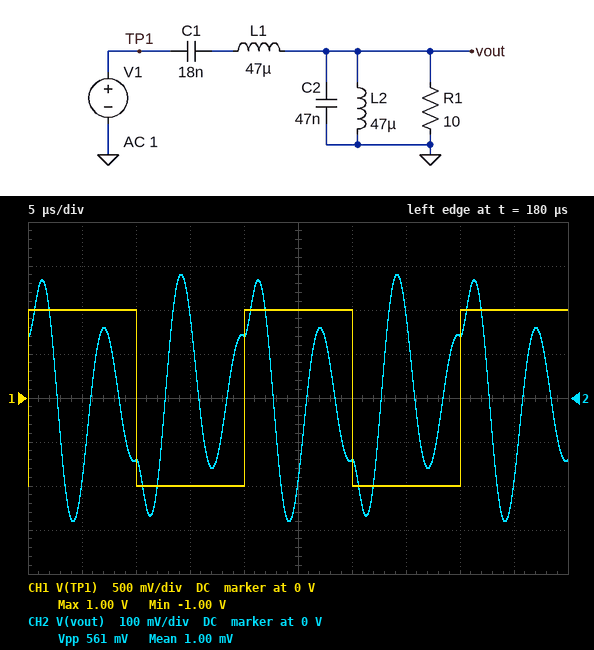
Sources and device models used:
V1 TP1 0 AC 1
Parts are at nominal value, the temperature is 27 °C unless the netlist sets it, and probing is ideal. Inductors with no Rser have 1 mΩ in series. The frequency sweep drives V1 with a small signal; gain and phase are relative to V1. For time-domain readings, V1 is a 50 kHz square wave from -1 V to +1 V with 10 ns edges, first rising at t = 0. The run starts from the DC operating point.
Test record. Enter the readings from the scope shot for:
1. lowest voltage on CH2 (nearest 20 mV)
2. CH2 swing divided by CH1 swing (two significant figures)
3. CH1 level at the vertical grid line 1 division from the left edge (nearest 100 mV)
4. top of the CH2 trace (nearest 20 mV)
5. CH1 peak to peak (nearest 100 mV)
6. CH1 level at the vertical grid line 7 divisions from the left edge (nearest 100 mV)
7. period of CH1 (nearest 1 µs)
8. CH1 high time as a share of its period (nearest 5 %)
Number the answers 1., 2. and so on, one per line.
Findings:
1. -280 mV
2. 0.28
3. 1.0 V
4. 280 mV
5. 2.0 V
6. -1.0 V
7. 20 µs
8. 50 %
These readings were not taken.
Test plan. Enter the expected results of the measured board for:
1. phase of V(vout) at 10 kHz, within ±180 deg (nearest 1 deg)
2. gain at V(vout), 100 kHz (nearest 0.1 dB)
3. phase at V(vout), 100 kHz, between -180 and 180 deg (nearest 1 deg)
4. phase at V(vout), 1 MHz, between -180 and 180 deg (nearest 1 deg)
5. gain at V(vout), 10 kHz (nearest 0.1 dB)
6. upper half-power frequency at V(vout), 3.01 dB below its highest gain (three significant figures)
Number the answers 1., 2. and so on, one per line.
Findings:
1. 163 deg
2. -15.5 dB
3. 83 deg
4. -161 deg
5. -49.8 dB
6. 195 kHz
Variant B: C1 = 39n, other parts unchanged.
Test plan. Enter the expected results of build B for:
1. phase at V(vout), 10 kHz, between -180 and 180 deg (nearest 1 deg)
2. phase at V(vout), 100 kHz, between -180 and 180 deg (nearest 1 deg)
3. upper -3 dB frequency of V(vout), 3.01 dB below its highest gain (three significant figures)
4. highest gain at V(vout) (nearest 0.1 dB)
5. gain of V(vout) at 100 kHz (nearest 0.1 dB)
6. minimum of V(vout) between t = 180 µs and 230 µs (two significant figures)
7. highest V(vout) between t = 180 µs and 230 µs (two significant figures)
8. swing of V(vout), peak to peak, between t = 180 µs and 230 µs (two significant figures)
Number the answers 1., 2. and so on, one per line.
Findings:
1. 163 deg
2. 50 deg
3. 139 kHz
4. 0 dB
5. -3.4 dB
6. -330 mV
7. 330 mV
8. 660 mV
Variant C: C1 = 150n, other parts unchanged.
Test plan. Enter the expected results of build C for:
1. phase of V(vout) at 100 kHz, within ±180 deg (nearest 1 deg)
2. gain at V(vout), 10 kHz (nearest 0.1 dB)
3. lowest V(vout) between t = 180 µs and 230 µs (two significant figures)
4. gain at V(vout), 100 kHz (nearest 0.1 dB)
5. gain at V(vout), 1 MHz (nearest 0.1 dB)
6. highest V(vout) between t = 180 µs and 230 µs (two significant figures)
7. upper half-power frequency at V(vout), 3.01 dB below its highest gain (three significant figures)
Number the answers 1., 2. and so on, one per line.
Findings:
1. -60 deg
2. -30.9 dB
3. -1.5 V
4. -6.8 dB
5. -39.1 dB
6. 1.5 V
7. 69.9 kHz
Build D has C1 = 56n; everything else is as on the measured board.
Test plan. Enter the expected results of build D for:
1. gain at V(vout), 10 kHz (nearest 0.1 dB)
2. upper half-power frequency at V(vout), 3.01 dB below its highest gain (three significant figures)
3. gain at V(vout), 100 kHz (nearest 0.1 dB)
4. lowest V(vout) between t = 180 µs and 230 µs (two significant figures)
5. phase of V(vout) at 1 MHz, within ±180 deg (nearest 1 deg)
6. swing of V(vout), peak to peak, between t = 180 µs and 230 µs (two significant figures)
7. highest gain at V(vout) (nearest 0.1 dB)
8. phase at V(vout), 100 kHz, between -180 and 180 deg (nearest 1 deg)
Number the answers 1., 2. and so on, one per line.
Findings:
1. -39.8 dB
2. 118 kHz
3. -0.1 dB
4. -360 mV
5. -161 deg
6. 720 mV
7. 0 dB
8. -6 deg
